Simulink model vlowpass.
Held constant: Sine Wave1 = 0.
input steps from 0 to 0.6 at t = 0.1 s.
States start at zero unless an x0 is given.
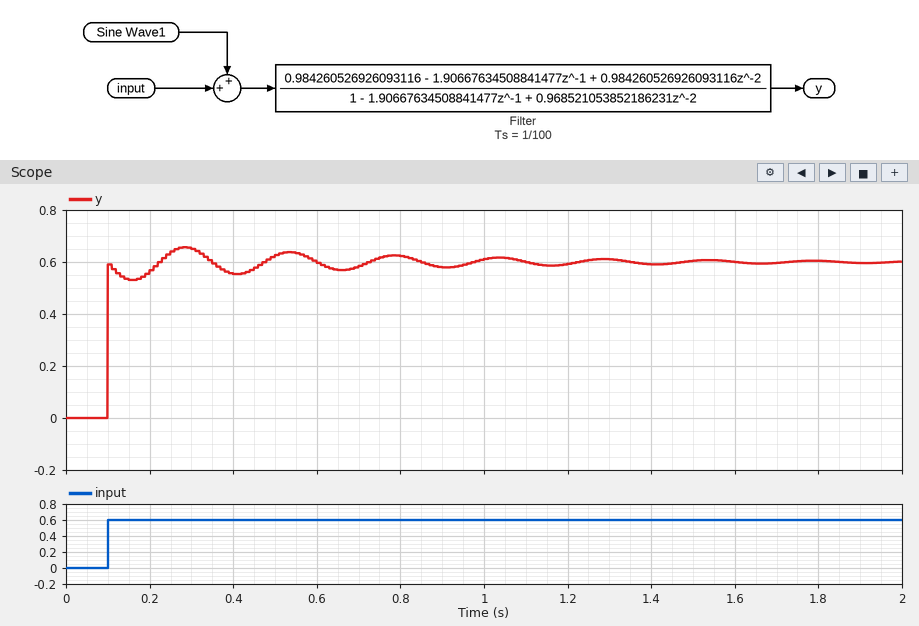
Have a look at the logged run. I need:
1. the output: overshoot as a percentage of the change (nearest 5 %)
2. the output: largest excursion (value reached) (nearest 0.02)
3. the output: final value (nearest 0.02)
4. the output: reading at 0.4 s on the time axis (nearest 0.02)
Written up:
10 %
0.66
0.60
0.56
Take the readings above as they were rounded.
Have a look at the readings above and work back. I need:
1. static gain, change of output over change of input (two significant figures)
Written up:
1.0
